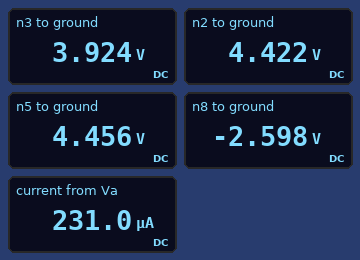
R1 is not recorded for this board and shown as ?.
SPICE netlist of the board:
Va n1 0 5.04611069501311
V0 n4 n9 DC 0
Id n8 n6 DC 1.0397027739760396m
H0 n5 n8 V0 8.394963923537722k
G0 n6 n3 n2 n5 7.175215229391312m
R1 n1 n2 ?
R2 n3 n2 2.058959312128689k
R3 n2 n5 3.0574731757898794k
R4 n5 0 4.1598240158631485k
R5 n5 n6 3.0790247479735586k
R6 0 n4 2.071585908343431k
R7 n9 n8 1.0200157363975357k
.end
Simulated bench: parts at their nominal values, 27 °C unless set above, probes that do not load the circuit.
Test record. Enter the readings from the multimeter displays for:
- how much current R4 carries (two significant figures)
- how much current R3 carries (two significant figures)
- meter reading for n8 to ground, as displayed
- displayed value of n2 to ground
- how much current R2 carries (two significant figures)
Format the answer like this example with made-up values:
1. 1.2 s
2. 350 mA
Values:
1. 1.1 mA
2. 11 µA
3. -2.598 V
4. 4.422 V
5. 240 µA
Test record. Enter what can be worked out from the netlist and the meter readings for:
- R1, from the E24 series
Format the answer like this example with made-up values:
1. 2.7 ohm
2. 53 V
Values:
1. 2.7 kΩ
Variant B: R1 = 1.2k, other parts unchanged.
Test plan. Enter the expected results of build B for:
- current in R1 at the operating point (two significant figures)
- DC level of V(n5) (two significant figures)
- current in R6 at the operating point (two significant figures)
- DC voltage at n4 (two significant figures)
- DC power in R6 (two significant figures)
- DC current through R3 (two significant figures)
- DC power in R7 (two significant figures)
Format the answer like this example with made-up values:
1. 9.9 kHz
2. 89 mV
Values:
1. 250 µA
2. 4.8 V
3. 900 µA
4. -1.9 V
5. 1.7 mW
6. 12 µA
7. 830 µW
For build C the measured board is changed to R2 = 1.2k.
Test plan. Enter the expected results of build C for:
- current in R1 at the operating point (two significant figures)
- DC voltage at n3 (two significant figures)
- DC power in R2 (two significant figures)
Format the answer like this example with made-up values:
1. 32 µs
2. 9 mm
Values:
1. 230 µA
2. 4.1 V
3. 70 µW
